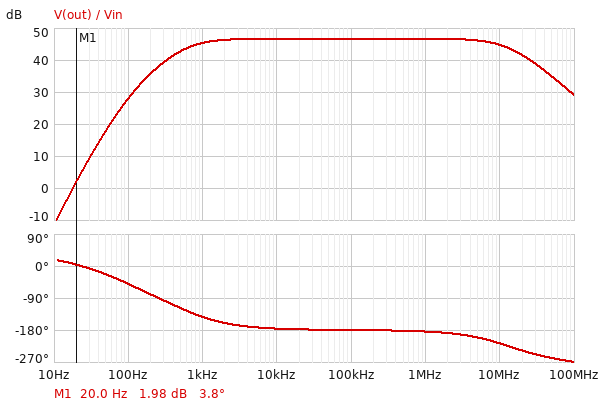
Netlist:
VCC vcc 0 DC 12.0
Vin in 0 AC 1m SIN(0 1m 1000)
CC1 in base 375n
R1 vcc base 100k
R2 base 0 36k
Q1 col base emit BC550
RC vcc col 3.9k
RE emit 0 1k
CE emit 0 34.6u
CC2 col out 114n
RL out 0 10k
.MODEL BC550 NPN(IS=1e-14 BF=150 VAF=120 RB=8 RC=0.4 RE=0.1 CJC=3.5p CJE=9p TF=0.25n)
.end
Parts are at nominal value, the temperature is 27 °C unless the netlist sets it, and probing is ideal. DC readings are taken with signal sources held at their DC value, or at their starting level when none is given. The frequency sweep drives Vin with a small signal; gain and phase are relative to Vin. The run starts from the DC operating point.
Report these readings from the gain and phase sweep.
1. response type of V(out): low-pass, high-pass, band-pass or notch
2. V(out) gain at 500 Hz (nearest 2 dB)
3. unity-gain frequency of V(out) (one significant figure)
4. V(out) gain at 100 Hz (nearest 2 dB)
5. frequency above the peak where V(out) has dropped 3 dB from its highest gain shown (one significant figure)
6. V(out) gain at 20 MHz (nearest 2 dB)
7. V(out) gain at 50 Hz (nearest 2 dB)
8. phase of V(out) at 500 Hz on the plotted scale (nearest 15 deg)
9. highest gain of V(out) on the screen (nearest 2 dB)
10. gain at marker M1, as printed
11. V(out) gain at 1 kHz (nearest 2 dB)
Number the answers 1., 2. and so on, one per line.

1. band-pass
2. 42 dB
3. 20 Hz
4. 28 dB
5. 10 MHz
6. 42 dB
7. 18 dB
8. -120 deg
9. 46 dB
10. 1.98 dB
11. 46 dB
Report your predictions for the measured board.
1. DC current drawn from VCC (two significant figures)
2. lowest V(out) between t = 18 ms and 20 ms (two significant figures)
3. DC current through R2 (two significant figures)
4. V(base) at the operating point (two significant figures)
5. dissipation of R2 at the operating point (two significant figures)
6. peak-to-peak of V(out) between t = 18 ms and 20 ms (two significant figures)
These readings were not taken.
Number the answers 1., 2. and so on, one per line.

1. 2.2 mA
2. -190 mV
3. 78 µA
4. 2.8 V
5. 220 µW
6. 370 mV
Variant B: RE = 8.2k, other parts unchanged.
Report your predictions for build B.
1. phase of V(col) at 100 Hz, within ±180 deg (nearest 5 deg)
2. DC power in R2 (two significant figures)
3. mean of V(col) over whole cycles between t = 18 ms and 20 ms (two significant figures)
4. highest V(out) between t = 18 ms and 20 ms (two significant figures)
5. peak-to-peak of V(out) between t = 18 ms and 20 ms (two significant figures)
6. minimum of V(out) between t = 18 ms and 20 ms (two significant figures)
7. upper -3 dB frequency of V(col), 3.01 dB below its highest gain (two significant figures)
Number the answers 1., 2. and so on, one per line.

1. -140 deg
2. 270 µW
3. 11 V
4. 32 mV
5. 65 mV
6. -33 mV
7. 33 MHz
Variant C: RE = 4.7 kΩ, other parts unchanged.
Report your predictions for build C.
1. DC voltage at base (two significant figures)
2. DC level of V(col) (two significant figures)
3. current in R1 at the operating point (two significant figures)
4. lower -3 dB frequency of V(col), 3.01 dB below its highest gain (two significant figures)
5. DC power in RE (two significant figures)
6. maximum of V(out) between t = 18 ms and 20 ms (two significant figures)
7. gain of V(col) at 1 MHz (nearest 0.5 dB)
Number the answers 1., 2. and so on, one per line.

1. 3.1 V
2. 10 V
3. 89 µA
4. 110 Hz
5. 1.3 mW
6. 54 mV
7. 35.0 dB
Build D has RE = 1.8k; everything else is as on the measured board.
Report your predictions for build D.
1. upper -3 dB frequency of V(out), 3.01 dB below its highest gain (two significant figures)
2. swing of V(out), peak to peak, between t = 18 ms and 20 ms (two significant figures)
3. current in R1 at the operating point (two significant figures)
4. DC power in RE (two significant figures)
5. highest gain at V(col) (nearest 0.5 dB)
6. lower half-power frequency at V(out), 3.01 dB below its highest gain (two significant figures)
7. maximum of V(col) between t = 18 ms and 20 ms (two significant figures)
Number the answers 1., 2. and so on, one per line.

1. 22 MHz
2. 250 mV
3. 90 µA
4. 2.9 mW
5. 42.5 dB
6. 390 Hz
7. 7.2 V
